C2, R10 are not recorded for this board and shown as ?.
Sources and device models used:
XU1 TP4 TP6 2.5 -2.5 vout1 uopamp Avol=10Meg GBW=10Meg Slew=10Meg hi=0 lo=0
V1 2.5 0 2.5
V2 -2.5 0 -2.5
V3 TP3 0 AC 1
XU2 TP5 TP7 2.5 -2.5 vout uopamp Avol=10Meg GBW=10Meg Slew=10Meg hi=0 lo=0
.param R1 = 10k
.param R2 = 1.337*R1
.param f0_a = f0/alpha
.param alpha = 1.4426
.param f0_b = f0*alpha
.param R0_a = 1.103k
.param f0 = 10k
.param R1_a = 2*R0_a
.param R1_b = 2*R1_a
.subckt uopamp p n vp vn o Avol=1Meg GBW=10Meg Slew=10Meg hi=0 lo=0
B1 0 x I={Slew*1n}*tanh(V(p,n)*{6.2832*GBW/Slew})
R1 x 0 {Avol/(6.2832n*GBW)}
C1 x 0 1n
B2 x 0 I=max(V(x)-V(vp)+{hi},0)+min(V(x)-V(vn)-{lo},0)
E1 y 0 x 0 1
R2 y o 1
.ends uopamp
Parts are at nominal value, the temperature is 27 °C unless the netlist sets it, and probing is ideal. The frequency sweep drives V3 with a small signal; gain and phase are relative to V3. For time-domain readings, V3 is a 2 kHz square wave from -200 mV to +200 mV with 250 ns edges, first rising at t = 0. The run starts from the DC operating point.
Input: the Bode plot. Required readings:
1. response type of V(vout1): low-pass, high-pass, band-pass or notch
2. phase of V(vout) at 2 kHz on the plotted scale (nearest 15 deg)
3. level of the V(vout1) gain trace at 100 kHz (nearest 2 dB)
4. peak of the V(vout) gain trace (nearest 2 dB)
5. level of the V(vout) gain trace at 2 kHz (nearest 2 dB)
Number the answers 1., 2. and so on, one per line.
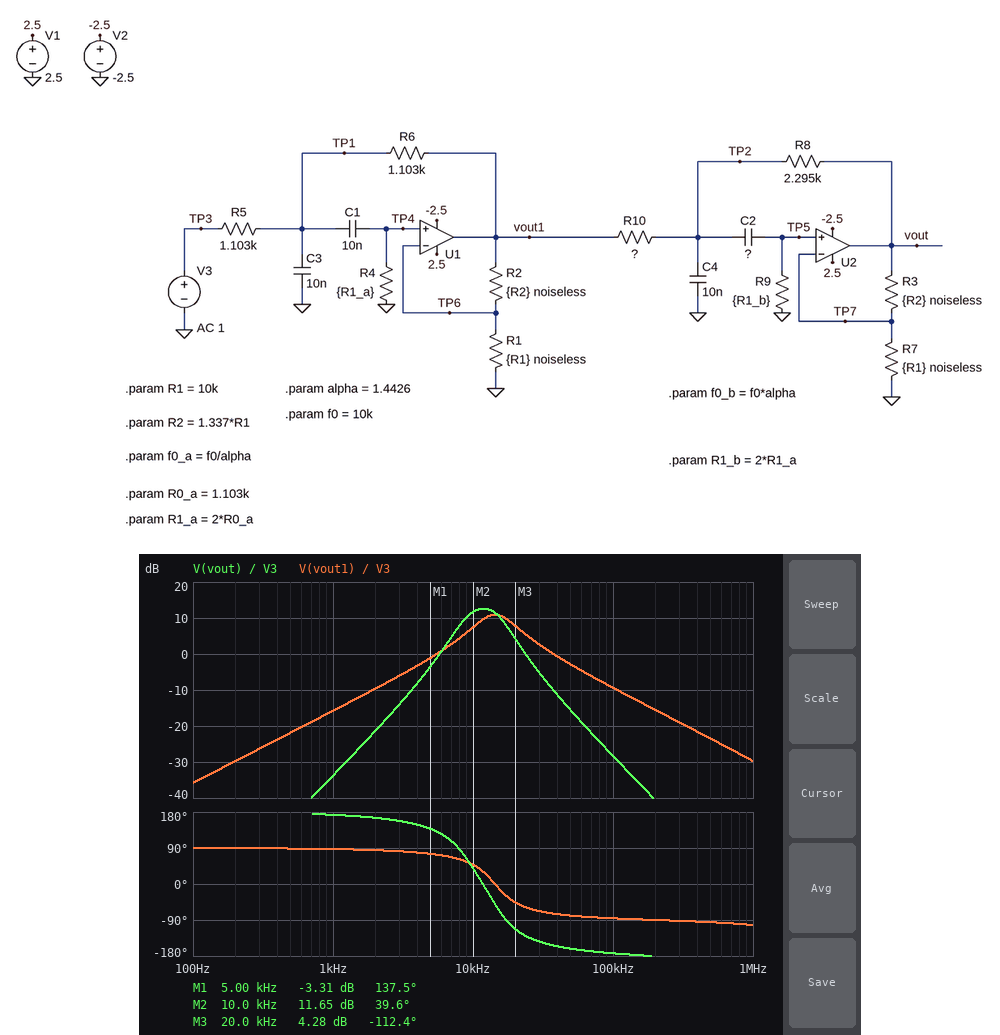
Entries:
1. band-pass
2. 165 deg
3. -10 dB
4. 12 dB
5. -22 dB
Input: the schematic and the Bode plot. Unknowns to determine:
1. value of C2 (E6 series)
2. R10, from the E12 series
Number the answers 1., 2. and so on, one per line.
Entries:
1. 4.7 nF
2. 3.3 kΩ
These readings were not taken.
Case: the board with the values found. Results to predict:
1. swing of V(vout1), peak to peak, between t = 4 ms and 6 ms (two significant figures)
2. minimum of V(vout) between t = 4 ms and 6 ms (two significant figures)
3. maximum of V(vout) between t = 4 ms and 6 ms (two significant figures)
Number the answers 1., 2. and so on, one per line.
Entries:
1. 1.2 V
2. -480 mV
3. 480 mV
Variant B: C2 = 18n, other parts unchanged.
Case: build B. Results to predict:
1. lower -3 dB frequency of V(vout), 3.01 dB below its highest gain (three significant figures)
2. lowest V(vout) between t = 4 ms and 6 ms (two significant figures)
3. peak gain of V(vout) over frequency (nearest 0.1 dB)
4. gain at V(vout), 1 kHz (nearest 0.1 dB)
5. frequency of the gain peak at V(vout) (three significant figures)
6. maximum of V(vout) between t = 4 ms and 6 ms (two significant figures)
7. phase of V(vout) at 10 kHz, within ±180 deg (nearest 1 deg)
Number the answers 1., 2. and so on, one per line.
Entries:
1. 4.42 kHz
2. -780 mV
3. 18.5 dB
4. -21.8 dB
5. 4.93 kHz
6. 780 mV
7. -33 deg
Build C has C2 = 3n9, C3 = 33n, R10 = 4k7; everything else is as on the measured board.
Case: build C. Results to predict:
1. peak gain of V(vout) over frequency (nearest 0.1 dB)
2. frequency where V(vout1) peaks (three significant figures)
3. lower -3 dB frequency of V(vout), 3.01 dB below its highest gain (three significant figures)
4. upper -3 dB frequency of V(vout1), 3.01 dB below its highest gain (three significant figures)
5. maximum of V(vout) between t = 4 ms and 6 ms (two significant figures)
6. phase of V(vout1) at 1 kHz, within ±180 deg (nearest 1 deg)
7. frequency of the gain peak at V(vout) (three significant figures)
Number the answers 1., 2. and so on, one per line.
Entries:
1. 2.8 dB
2. 7.93 kHz
3. 6.83 kHz
4. 12.8 kHz
5. 150 mV
6. 83 deg
7. 9.11 kHz
